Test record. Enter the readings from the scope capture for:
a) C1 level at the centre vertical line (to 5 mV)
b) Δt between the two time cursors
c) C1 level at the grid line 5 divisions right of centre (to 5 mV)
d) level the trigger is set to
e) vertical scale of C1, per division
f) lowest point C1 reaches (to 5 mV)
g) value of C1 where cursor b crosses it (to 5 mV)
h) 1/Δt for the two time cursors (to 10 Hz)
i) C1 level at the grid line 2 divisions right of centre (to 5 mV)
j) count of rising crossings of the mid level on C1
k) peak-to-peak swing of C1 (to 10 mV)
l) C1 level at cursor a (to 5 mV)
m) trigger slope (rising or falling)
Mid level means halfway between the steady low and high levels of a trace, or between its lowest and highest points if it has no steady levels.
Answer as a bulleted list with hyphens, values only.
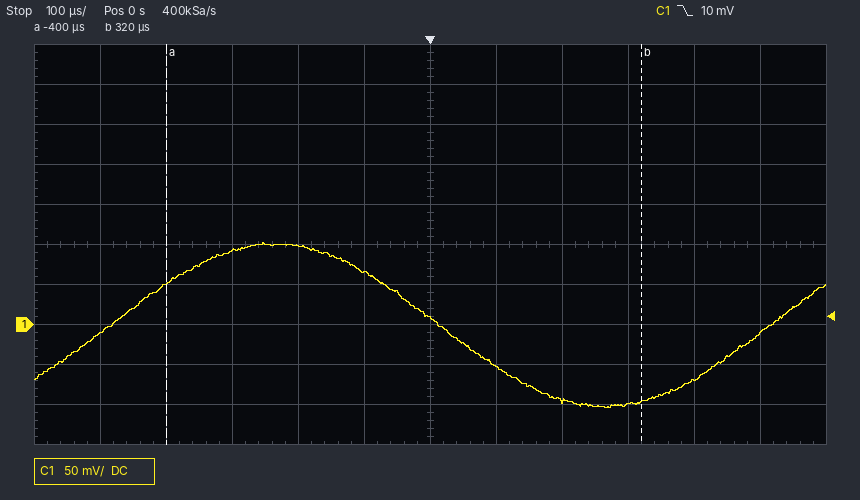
- 10 mV
- 720 µs
- -10 mV
- 10 mV
- 50 mV
- -105 mV
- -95 mV
- 1.39 kHz
- -95 mV
- 2
- 210 mV
- 50 mV
- falling
